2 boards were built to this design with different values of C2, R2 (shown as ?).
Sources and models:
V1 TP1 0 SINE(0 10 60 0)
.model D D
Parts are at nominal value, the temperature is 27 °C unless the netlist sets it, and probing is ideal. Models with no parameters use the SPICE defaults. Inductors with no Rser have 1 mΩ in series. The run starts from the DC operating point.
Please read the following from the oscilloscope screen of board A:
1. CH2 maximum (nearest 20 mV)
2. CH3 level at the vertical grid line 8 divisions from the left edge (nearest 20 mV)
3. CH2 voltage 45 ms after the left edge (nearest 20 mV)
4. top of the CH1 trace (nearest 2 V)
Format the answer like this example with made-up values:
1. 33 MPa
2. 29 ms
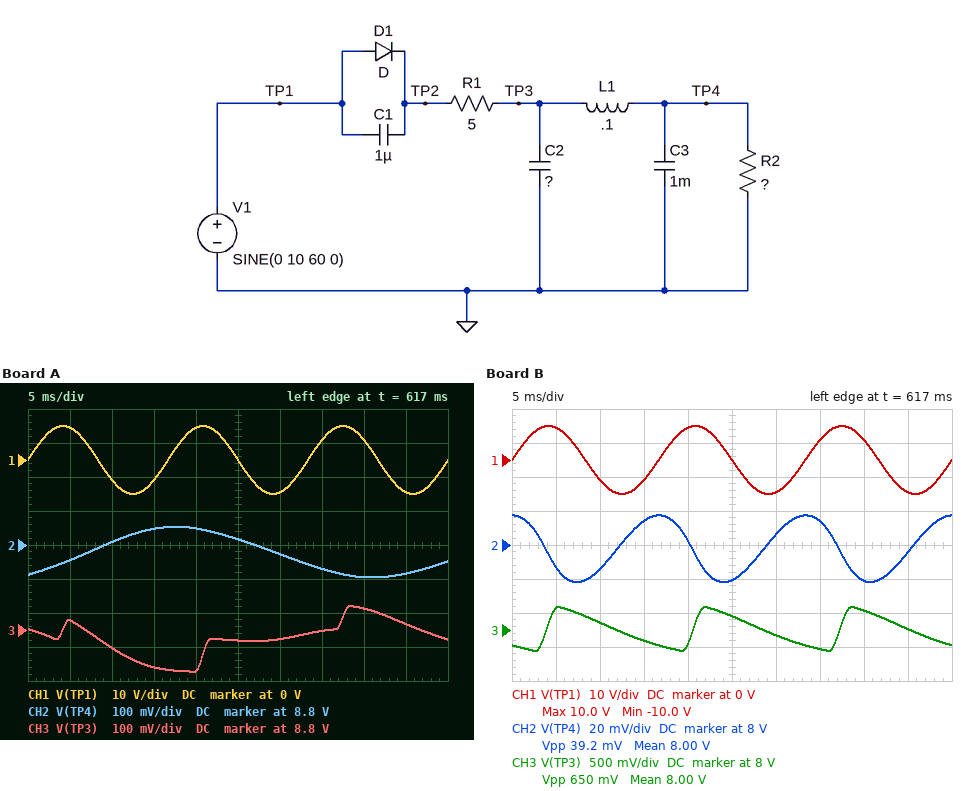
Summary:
1. 8.86 V
2. 8.86 V
3. 8.72 V
4. 10 V
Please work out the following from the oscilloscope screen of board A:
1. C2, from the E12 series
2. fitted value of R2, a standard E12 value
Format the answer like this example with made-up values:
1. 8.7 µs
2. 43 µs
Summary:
1. 1.2 mF
2. 1.5 kΩ
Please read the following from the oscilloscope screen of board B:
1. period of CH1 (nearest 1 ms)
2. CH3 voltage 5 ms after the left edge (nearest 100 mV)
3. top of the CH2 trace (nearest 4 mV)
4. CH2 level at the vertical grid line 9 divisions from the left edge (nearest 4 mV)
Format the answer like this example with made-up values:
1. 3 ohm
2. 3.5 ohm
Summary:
1. 17 ms
2. 8.3 V
3. 8.016 V
4. 7.996 V
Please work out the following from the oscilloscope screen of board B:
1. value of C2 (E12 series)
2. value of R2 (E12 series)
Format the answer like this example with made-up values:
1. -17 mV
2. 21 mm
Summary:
1. 560 µF
2. 330 Ω
